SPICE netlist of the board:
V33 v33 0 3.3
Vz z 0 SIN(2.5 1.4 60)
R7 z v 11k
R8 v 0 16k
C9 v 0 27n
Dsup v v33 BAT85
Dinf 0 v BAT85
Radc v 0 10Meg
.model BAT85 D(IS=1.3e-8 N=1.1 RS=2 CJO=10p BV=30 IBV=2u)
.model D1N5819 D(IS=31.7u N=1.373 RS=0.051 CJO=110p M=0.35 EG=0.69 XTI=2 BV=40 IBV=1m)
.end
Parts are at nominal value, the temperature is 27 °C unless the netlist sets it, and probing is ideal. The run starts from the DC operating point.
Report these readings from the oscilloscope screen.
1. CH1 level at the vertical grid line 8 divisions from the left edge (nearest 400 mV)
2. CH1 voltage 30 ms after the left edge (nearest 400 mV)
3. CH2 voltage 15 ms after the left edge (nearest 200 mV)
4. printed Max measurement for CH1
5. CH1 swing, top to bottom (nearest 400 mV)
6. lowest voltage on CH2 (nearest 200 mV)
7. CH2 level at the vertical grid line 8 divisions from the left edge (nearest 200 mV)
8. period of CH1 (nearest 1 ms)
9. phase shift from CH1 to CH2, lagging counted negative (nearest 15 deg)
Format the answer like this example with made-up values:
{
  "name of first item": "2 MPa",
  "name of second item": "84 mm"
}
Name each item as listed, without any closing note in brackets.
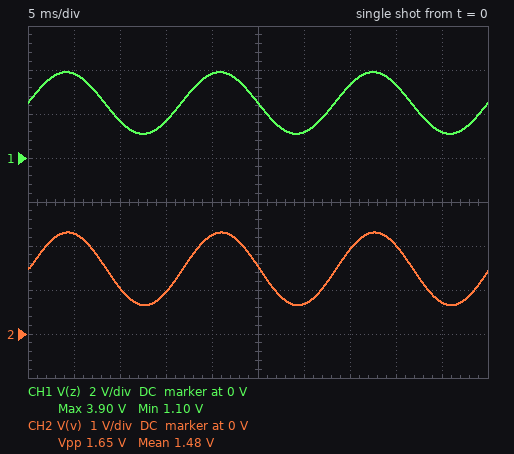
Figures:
{
  "CH1 level at the vertical grid line 8 divisions from the left edge": "3.2 V",
  "CH1 voltage 30 ms after the left edge": "1.2 V",
  "CH2 voltage 15 ms after the left edge": "1.0 V",
  "printed Max measurement for CH1": "3.90 V",
  "CH1 swing, top to bottom": "2.8 V",
  "lowest voltage on CH2": "600 mV",
  "CH2 level at the vertical grid line 8 divisions from the left edge": "2.0 V",
  "period of CH1": "17 ms",
  "phase shift from CH1 to CH2, lagging counted negative": "0 deg"
}
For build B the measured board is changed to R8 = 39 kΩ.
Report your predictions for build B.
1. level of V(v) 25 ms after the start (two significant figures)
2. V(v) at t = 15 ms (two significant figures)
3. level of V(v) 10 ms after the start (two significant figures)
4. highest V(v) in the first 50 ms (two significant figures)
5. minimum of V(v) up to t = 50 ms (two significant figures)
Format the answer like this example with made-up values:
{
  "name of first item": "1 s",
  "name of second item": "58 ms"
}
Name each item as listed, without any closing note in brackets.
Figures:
{
  "level of V(v) 25 ms after the start": "2.0 V",
  "V(v) at t = 15 ms": "1.2 V",
  "level of V(v) 10 ms after the start": "1.4 V",
  "highest V(v) in the first 50 ms": "3.0 V",
  "minimum of V(v) up to t = 50 ms": "860 mV"
}
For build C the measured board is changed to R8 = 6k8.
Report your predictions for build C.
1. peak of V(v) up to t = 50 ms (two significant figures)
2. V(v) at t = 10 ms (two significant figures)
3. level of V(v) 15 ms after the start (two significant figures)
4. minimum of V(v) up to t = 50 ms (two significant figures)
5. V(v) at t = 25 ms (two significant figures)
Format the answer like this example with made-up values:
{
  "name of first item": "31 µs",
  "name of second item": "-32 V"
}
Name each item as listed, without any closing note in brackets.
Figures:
{
  "peak of V(v) up to t = 50 ms": "1.5 V",
  "V(v) at t = 10 ms": "660 mV",
  "level of V(v) 15 ms after the start": "620 mV",
  "minimum of V(v) up to t = 50 ms": "420 mV",
  "V(v) at t = 25 ms": "980 mV"
}
